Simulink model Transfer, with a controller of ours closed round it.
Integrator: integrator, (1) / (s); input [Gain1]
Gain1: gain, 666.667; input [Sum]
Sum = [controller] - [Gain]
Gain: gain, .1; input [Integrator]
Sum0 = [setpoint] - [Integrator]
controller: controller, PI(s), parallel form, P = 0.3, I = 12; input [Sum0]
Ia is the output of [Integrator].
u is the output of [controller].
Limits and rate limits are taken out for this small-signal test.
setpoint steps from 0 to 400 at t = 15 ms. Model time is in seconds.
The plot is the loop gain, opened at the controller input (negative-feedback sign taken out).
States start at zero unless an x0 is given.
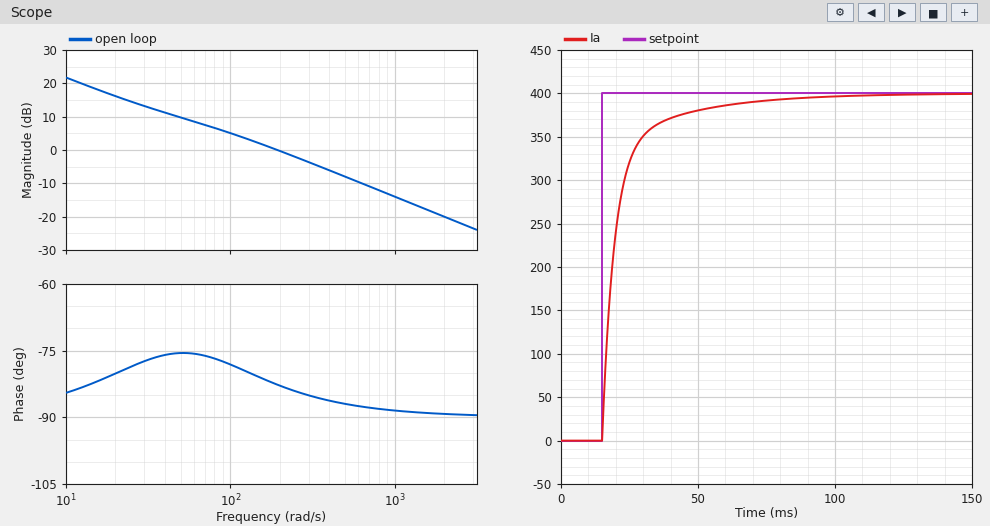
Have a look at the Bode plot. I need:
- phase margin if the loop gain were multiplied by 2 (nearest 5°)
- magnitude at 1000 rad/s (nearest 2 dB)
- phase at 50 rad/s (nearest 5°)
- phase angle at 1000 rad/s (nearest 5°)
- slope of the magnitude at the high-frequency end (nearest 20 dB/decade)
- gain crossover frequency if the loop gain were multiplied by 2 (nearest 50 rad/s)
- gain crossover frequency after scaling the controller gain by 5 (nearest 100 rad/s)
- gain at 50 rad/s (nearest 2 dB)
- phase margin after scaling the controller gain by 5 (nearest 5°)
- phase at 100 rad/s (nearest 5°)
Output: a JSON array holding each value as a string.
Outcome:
["95°", "-14 dB", "-75°", "-90°", "-20 dB/decade", "400 rad/s", "1000 rad/s", "10 dB", "90°", "-80°"]
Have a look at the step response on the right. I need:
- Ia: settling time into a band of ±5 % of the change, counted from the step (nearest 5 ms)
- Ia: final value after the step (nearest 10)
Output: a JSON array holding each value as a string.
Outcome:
["35 ms", "400"]
